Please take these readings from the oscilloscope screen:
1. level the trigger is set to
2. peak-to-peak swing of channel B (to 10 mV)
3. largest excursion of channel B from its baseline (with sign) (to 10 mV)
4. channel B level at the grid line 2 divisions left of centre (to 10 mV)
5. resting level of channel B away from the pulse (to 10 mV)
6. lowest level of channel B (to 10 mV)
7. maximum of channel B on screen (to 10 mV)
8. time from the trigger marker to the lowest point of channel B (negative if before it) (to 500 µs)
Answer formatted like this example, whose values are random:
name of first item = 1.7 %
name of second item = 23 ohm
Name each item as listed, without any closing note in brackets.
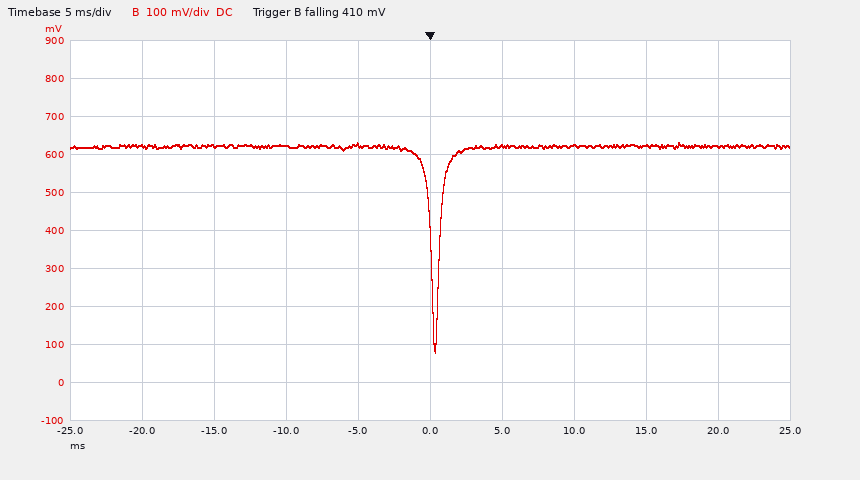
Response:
level the trigger is set to = 410 mV
peak-to-peak swing of channel B = 550 mV
largest excursion of channel B from its baseline (with sign) = -540 mV
channel B level at the grid line 2 divisions left of centre = 620 mV
resting level of channel B away from the pulse = 620 mV
lowest level of channel B = 80 mV
maximum of channel B on screen = 630 mV
time from the trigger marker to the lowest point of channel B (negative if before it) = +500 µs
